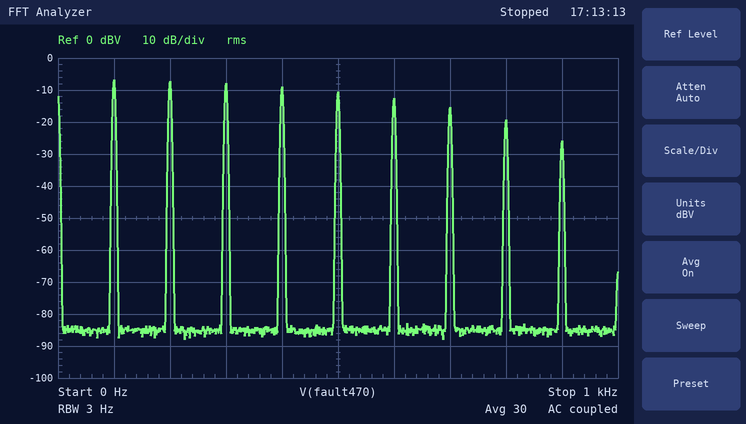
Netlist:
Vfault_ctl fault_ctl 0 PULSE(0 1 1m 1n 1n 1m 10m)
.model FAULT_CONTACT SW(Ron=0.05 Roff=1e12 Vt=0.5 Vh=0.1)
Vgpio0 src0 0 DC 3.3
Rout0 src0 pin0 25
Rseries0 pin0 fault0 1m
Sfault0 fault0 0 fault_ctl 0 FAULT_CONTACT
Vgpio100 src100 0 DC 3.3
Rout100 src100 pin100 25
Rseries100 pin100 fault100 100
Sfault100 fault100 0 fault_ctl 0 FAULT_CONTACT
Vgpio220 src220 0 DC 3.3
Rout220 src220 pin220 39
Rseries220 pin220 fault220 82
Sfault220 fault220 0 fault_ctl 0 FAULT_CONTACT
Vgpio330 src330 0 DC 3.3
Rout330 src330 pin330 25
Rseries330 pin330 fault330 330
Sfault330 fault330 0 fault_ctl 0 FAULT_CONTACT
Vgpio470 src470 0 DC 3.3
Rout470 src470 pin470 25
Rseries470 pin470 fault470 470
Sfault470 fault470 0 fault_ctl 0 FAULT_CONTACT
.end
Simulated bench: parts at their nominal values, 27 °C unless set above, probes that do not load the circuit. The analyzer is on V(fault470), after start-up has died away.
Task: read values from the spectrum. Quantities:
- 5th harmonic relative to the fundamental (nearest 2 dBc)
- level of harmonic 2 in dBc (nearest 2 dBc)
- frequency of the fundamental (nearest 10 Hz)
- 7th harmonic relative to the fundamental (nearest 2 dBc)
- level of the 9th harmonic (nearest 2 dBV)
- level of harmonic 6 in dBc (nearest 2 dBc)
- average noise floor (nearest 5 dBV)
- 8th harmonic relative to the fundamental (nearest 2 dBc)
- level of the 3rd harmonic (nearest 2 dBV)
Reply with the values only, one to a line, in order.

-4 dBc
0 dBc
100 Hz
-8 dBc
-26 dBV
-6 dBc
-85 dBV
-12 dBc
-8 dBV
